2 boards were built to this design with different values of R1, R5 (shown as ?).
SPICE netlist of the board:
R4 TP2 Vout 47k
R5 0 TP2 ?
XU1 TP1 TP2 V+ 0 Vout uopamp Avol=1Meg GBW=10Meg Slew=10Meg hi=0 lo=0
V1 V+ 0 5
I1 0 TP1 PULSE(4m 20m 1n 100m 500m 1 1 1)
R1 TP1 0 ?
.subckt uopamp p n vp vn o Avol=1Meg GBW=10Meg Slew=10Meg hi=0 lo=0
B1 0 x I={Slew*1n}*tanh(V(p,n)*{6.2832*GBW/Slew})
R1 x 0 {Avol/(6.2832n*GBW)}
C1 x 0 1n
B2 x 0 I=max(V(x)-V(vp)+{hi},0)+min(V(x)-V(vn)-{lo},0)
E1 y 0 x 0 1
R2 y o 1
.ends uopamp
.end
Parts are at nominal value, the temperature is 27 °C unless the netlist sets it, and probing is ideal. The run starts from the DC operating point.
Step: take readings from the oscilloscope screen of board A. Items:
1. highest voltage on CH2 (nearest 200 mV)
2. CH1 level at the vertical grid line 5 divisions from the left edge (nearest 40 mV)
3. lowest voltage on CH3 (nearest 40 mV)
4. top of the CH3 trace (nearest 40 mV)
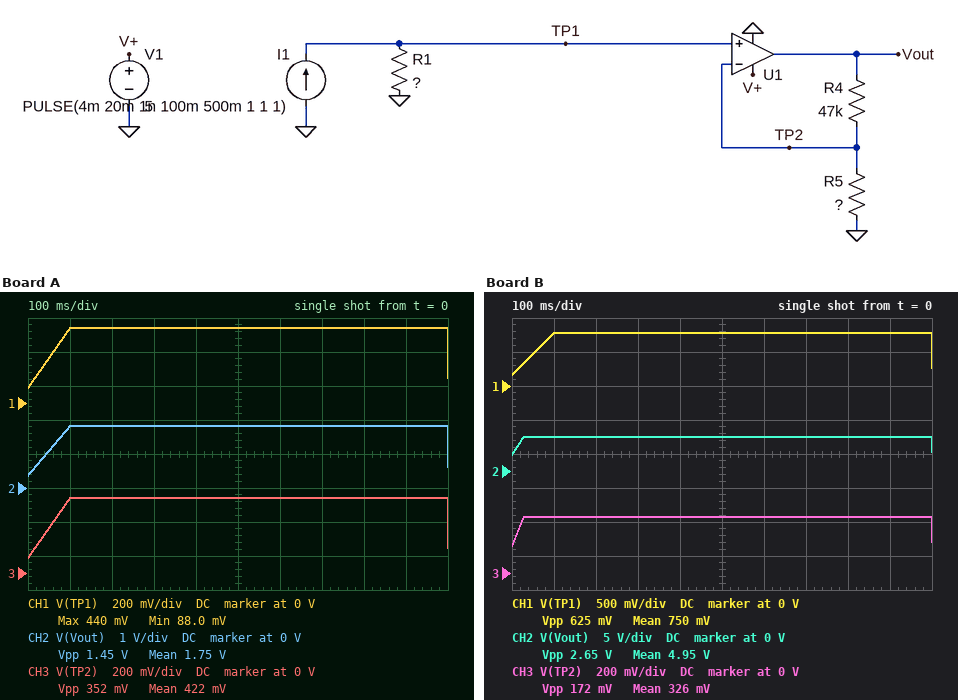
1.8 V
440 mV
80 mV
440 mV
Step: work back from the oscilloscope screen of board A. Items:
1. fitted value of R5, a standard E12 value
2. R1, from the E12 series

15 kΩ
22 Ω
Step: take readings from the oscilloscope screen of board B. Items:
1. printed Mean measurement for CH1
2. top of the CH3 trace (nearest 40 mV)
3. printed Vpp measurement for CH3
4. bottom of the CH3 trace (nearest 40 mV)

750 mV
320 mV
172 mV
160 mV
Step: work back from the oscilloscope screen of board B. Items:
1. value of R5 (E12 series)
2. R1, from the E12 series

3.3 kΩ
39 Ω
